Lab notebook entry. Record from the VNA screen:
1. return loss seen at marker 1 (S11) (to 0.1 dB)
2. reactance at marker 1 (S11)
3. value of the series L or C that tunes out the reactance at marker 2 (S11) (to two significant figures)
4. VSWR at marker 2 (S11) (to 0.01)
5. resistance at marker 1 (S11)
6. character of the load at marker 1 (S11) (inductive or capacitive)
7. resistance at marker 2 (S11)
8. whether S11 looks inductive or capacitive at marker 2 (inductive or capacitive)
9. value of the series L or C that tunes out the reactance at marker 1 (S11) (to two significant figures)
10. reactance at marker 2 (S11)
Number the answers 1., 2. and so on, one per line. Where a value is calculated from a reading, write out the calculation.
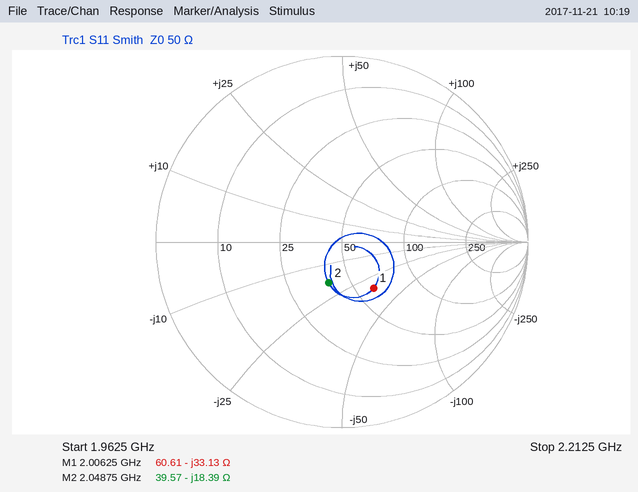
1. 10.4 dB
2. -33.13 Ω
3. L = 18.39 Ω/(2π × 2.04875 GHz) ≈ 1.4 nH
4. 1.60
5. 60.61 Ω
6. capacitive
7. 39.57 Ω
8. capacitive
9. L = 33.13 Ω/(2π × 2.00625 GHz) ≈ 2.6 nH
10. -18.39 Ω
